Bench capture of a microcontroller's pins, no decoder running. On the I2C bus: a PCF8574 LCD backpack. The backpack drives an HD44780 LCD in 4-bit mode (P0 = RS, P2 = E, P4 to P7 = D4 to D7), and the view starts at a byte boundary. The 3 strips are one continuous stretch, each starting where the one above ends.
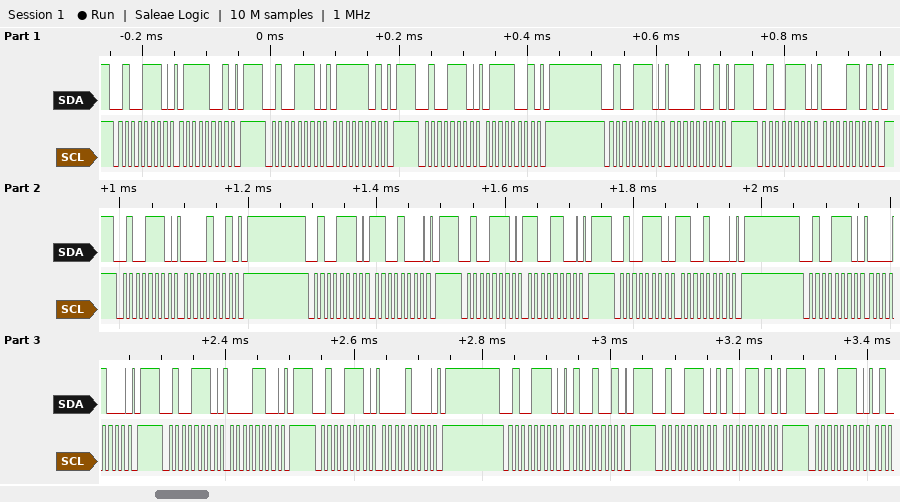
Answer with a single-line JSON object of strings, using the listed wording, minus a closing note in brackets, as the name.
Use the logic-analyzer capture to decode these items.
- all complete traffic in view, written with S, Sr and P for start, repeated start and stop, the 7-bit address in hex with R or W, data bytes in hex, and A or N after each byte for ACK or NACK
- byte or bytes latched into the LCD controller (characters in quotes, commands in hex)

{"all complete traffic in view, written with S, Sr and P for start, repeated start and stop, the 7-bit address in hex with R or W, data bytes in hex, and A or N after each byte for ACK or NACK": "S 27W A 79 A P S 27W A 7D A P S 27W A 79 A P S 27W A 09 A P S 27W A 0D A P S 27W A 09 A P S 27W A C8 A P S 27W A CC A P S 27W A C8 A P S 27W A 08 A P S 27W A 0C A P S 27W A 08 A P S 27W A 49 A P S 27W A 4D A P S 27W A", "byte or bytes latched into the LCD controller": "'p' 0xC0"}
